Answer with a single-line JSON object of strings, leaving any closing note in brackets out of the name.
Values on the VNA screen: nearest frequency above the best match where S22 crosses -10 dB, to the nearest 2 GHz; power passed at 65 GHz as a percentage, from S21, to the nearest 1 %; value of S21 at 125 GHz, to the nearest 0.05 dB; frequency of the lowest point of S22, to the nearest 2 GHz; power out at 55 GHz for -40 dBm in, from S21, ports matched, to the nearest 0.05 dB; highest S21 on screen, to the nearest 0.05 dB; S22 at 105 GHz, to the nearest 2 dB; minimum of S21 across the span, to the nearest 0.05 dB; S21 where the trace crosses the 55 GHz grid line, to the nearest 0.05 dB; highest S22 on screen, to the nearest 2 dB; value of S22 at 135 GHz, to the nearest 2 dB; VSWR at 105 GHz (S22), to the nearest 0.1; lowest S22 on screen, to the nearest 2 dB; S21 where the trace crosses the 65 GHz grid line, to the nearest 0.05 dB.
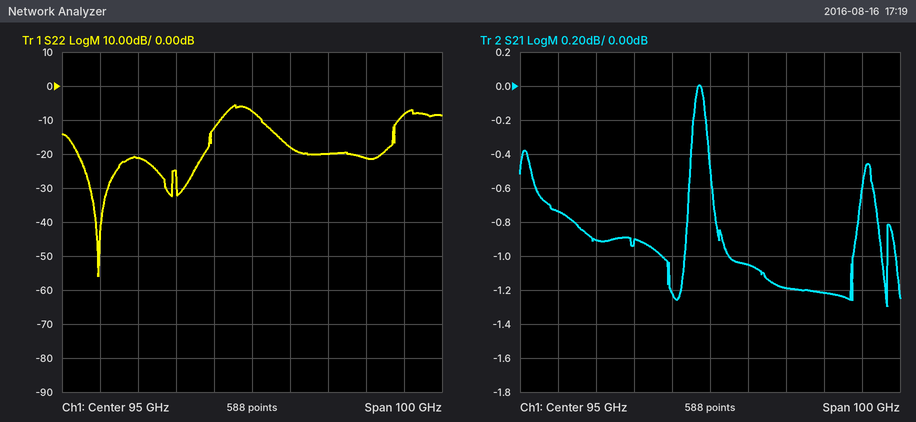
{"nearest frequency above the best match where S22 crosses -10 dB, to the nearest 2 GHz": "86 GHz", "power passed at 65 GHz as a percentage, from S21, to the nearest 1 %": "81 %", "value of S21 at 125 GHz, to the nearest 0.05 dB": "-1.20 dB", "frequency of the lowest point of S22, to the nearest 2 GHz": "54 GHz", "power out at 55 GHz for -40 dBm in, from S21, ports matched, to the nearest 0.05 dB": "-40.75 dBm", "highest S21 on screen, to the nearest 0.05 dB": "0.00 dB", "S22 at 105 GHz, to the nearest 2 dB": "-18 dB", "minimum of S21 across the span, to the nearest 0.05 dB": "-1.30 dB", "S21 where the trace crosses the 55 GHz grid line, to the nearest 0.05 dB": "-0.75 dB", "highest S22 on screen, to the nearest 2 dB": "-6 dB", "value of S22 at 135 GHz, to the nearest 2 dB": "-8 dB", "VSWR at 105 GHz (S22), to the nearest 0.1": "1.3", "lowest S22 on screen, to the nearest 2 dB": "-56 dB", "S21 where the trace crosses the 65 GHz grid line, to the nearest 0.05 dB": "-0.90 dB"}
